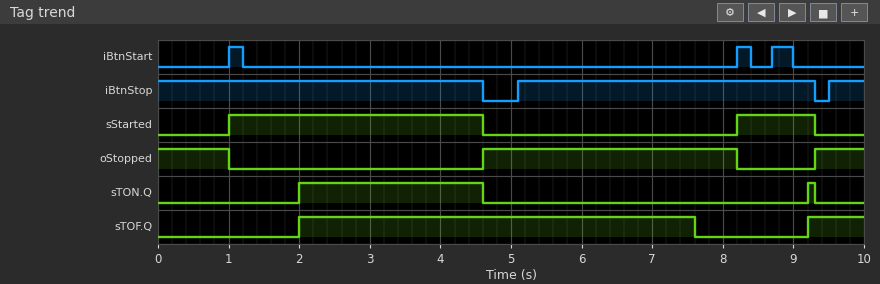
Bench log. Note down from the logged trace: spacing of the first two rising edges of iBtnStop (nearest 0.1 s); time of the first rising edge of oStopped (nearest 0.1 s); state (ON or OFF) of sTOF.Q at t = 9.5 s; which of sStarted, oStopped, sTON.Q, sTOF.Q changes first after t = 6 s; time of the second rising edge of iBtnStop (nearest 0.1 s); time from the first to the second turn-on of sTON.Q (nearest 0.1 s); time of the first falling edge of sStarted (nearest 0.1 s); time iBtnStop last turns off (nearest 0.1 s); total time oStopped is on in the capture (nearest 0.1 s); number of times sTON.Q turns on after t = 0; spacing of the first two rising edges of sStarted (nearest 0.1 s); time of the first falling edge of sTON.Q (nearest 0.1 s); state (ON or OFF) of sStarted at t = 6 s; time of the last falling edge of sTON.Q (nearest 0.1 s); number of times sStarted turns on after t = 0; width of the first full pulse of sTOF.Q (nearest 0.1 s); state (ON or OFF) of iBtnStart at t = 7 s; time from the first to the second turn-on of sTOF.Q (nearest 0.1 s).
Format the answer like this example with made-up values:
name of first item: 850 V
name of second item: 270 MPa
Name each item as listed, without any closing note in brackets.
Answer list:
spacing of the first two rising edges of iBtnStop: 4.4 s
time of the first rising edge of oStopped: 4.6 s
state (ON or OFF) of sTOF.Q at t = 9.5 s: ON
which of sStarted, oStopped, sTON.Q, sTOF.Q changes first after t = 6 s: sTOF.Q
time of the second rising edge of iBtnStop: 9.5 s
time from the first to the second turn-on of sTON.Q: 7.2 s
time of the first falling edge of sStarted: 4.6 s
time iBtnStop last turns off: 9.3 s
total time oStopped is on in the capture: 5.3 s
number of times sTON.Q turns on after t = 0: 2
spacing of the first two rising edges of sStarted: 7.2 s
time of the first falling edge of sTON.Q: 4.6 s
state (ON or OFF) of sStarted at t = 6 s: OFF
time of the last falling edge of sTON.Q: 9.3 s
number of times sStarted turns on after t = 0: 2
width of the first full pulse of sTOF.Q: 5.6 s
state (ON or OFF) of iBtnStart at t = 7 s: OFF
time from the first to the second turn-on of sTOF.Q: 7.2 s
